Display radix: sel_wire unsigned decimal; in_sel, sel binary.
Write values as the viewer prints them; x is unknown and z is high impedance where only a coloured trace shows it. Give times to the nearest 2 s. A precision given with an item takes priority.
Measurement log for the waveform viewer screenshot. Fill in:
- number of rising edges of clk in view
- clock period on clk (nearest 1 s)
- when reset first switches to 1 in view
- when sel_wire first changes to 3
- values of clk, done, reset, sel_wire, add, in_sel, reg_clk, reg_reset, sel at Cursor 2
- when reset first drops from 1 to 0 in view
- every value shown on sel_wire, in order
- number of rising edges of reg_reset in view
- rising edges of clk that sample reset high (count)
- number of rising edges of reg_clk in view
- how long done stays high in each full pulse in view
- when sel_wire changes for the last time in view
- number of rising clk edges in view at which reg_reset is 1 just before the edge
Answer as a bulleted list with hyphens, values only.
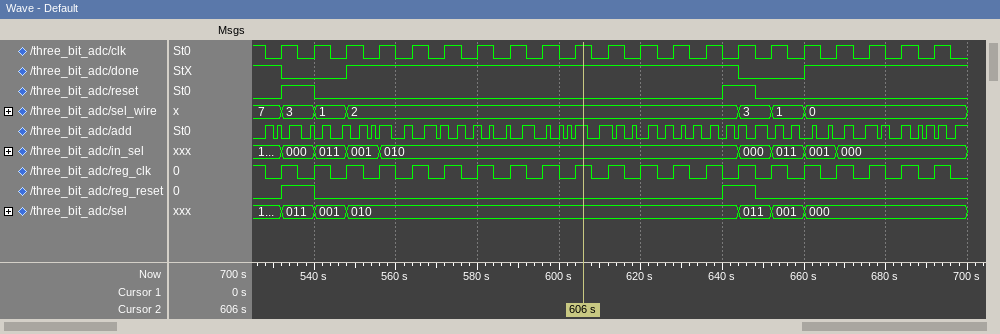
- 21
- 8 s
- 532 s
- 532 s
- clk=1, done=1, reset=0, sel_wire=2, add=1, in_sel=010, reg_clk=1, reg_reset=0, sel=010
- 540 s
- 7, 3, 1, 2, 3, 1, 0
- 2
- 2
- 21
- 96 s
- 660 s
- 2
